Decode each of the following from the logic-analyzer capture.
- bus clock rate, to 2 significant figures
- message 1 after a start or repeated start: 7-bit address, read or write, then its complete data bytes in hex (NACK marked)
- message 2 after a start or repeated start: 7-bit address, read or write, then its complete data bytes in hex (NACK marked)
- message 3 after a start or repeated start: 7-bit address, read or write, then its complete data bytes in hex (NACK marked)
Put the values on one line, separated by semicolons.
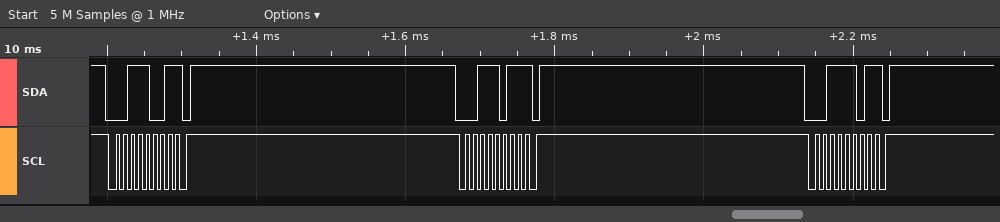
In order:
100 kHz; 0x1C read NACK; 0x1D read NACK; 0x1E read NACK
